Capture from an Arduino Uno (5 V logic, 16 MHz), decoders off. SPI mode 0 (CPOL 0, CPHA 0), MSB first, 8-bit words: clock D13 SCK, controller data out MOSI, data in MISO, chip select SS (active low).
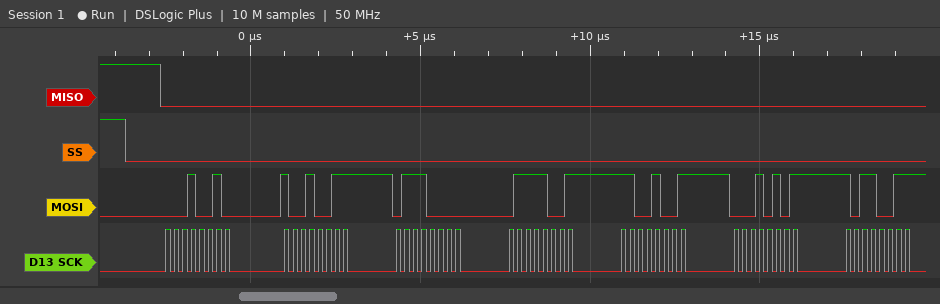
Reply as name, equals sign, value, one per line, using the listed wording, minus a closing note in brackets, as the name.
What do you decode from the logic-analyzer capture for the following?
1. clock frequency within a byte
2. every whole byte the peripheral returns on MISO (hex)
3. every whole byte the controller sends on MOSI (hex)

clock frequency within a byte = 4 MHz
every whole byte the peripheral returns on MISO = 00 00 00 00 00 00 00
every whole byte the controller sends on MOSI = 12 93 70 79 C9 15 B3
